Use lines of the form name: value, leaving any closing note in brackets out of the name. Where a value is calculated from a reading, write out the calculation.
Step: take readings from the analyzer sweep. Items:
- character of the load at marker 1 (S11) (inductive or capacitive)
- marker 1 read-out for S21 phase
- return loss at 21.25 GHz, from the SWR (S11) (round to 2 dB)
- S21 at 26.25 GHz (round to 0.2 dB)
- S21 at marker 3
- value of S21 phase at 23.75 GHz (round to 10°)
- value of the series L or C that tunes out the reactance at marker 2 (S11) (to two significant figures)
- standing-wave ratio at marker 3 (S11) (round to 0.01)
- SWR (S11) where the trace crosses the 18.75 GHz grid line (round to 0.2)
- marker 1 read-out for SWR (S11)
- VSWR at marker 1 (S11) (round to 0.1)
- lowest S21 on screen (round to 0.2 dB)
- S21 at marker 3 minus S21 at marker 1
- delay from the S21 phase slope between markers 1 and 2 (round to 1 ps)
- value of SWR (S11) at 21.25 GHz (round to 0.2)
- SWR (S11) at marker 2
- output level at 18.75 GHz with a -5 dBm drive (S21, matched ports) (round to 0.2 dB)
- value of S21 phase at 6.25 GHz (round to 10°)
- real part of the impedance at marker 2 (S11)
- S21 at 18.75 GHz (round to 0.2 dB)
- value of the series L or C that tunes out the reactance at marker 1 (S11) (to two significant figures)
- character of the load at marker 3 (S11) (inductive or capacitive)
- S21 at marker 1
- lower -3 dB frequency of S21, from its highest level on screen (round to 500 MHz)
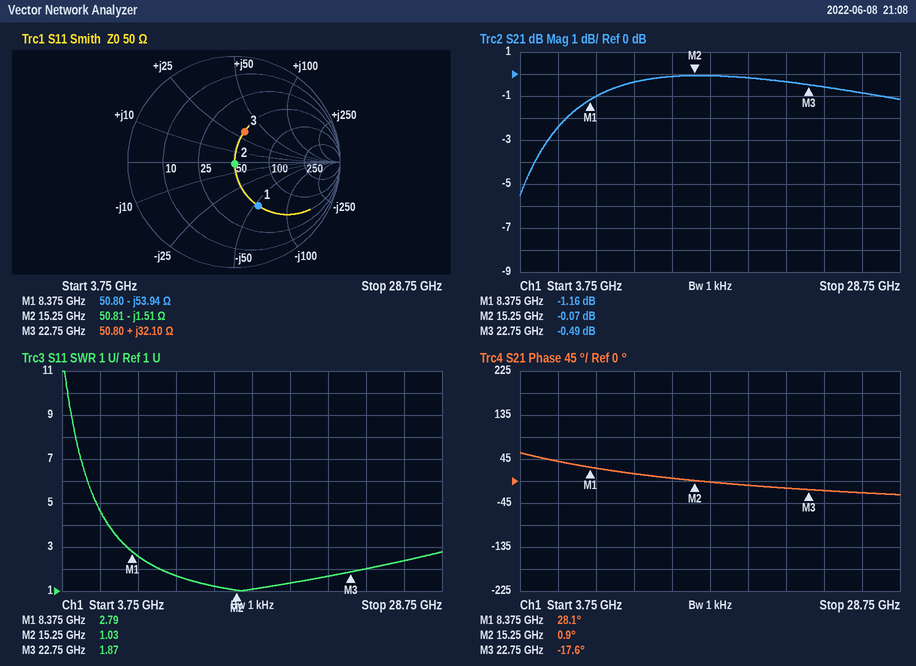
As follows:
character of the load at marker 1 (S11): capacitive
marker 1 read-out for S21 phase: 28.1°
return loss at 21.25 GHz, from the SWR (S11): −20 log10((1.6 − 1)/(1.6 + 1)) ≈ 12.7 dB, so 12 dB to the nearest 2 dB
S21 at 26.25 GHz: -0.8 dB
S21 at marker 3: -0.49 dB
value of S21 phase at 23.75 GHz: -20°
value of the series L or C that tunes out the reactance at marker 2 (S11): L = 1.51 Ω/(2π × 15.25 GHz) ≈ 16 pH
standing-wave ratio at marker 3 (S11): 1.87
SWR (S11) where the trace crosses the 18.75 GHz grid line: 1.4
marker 1 read-out for SWR: 2.79
VSWR at marker 1 (S11): 2.8
lowest S21 on screen: -5.6 dB
S21 at marker 3 minus S21 at marker 1: -0.49 − (-1.16) = 0.67 dB
delay from the S21 phase slope between markers 1 and 2: −(0.9° − (28.1°))/(360° × 6.875 GHz) ≈ 11 ps
value of SWR (S11) at 21.25 GHz: 1.6
SWR (S11) at marker 2: 1.03
output level at 18.75 GHz with a -5 dBm drive (S21, matched ports): -5 dBm + (-0.2 dB) = -5.2 dBm
value of S21 phase at 6.25 GHz: 40°
real part of the impedance at marker 2: 50.81 Ω
S21 at 18.75 GHz: -0.2 dB
value of the series L or C that tunes out the reactance at marker 1 (S11): L = 53.94 Ω/(2π × 8.375 GHz) ≈ 1.0 nH
character of the load at marker 3 (S11): inductive
S21 at marker 1: -1.16 dB
lower -3 dB frequency of S21, from its highest level on screen: 5.5 GHz
